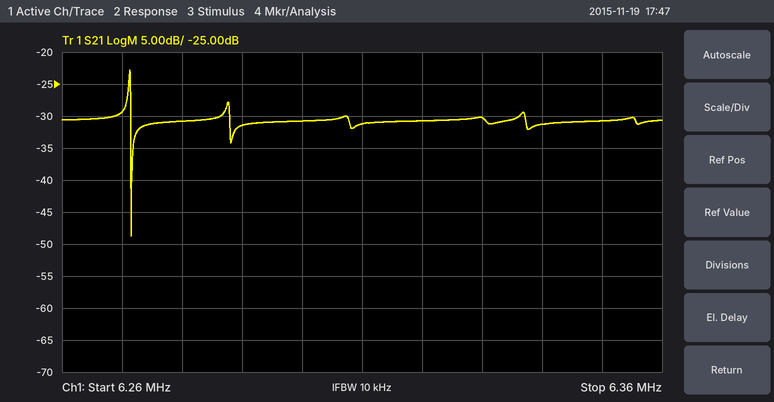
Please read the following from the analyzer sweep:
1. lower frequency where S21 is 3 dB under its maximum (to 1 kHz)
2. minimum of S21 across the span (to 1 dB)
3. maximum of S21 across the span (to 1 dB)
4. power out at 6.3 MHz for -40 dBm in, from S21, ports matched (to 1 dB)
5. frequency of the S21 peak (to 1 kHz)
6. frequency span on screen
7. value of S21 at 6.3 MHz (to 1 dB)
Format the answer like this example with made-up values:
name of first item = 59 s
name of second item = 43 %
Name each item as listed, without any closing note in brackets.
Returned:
lower frequency where S21 is 3 dB under its maximum = 6.271 MHz
minimum of S21 across the span = -49 dB
maximum of S21 across the span = -23 dB
power out at 6.3 MHz for -40 dBm in, from S21, ports matched = -71 dBm
frequency of the S21 peak = 6.271 MHz
frequency span on screen = 100 kHz
value of S21 at 6.3 MHz = -31 dB
